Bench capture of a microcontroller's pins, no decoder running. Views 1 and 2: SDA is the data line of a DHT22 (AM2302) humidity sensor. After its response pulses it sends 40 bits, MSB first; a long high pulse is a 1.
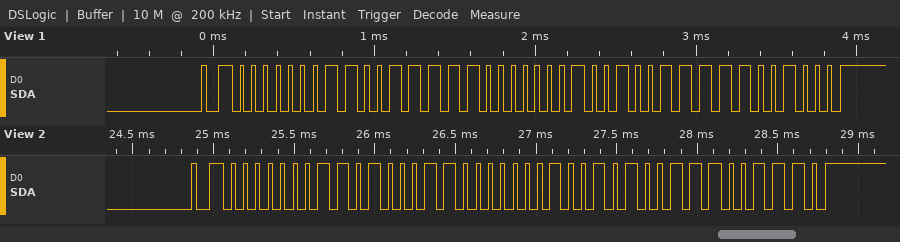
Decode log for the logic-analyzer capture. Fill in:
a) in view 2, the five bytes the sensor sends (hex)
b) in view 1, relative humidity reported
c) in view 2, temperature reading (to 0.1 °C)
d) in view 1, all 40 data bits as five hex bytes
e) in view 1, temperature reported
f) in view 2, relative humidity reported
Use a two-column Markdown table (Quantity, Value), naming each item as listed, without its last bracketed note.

| Quantity | Value |
|---|---|
| in view 2, the five bytes the sensor sends | 01 A3 01 29 CE |
| in view 1, relative humidity reported | 41.5 % |
| in view 2, temperature reading | 29.7 °C |
| in view 1, all 40 data bits as five hex bytes | 01 9F 01 27 C8 |
| in view 1, temperature reported | 29.5 °C |
| in view 2, relative humidity reported | 41.9 % |
